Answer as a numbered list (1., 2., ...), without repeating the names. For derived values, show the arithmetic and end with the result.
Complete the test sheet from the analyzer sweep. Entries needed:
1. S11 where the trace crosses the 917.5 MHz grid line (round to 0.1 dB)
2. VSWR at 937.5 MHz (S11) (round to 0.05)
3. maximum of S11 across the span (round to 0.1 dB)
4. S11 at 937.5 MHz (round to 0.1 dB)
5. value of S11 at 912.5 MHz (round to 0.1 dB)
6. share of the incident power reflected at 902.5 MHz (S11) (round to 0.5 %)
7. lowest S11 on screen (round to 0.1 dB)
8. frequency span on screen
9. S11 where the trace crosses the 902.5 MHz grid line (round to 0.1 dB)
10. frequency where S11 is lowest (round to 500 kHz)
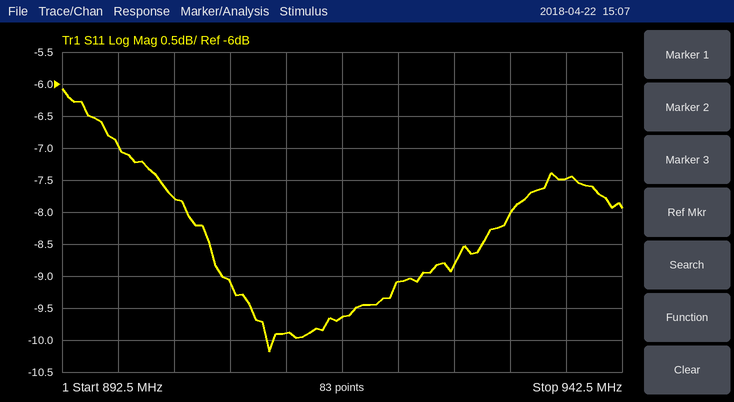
1. -9.6 dB
2. |Γ| = 10^(-7.5/20) = 0.4217; VSWR = (1 + 0.4217)/(1 − 0.4217) ≈ 2.46, so 2.45 to the nearest 0.05
3. -6.1 dB
4. -7.5 dB
5. -9.9 dB
6. 10^(-7.8/10) ≈ 16.6 %, so 16.5 % to the nearest 0.5 %
7. -10.2 dB
8. 50 MHz
9. -7.8 dB
10. 911.0 MHz
